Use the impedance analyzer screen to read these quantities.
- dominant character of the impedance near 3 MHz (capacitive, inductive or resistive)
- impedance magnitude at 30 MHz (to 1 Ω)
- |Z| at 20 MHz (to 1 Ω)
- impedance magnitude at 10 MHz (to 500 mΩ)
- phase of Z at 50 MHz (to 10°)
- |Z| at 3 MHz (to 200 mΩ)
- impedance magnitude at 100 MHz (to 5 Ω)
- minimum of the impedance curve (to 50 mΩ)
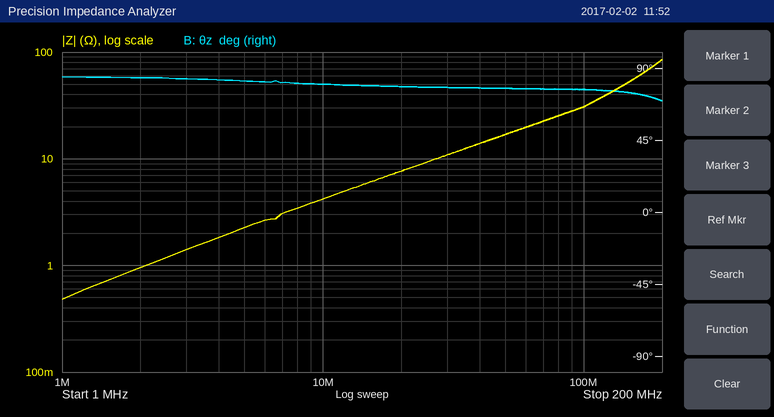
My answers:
inductive
11 Ω
8 Ω
4.0 Ω
80°
1.4 Ω
30 Ω
500 mΩ
